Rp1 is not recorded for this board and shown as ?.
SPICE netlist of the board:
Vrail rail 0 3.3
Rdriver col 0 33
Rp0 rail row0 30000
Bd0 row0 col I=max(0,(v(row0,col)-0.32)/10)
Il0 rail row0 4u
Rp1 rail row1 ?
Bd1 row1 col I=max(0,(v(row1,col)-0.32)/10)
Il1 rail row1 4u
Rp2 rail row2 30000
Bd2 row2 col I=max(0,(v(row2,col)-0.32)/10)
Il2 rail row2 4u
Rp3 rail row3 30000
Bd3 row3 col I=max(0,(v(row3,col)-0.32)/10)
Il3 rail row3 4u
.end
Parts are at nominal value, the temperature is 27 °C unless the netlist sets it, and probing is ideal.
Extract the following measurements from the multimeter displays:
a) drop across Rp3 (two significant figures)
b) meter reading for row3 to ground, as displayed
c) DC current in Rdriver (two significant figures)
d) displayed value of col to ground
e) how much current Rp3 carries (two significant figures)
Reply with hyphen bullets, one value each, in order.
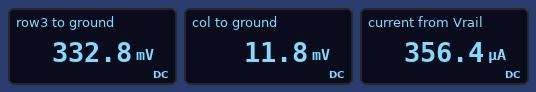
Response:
- 3.0 V
- 332.8 mV
- 360 µA
- 11.8 mV
- 99 µA
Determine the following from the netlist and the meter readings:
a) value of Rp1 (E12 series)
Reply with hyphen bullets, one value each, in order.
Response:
- 68 kΩ
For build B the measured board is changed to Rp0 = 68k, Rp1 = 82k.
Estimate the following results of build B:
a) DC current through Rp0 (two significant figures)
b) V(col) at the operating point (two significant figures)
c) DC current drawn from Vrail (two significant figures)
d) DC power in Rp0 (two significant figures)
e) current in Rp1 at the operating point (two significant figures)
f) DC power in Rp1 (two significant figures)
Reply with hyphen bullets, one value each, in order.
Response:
- 44 µA
- 9.7 mV
- 290 µA
- 130 µW
- 36 µA
- 110 µW
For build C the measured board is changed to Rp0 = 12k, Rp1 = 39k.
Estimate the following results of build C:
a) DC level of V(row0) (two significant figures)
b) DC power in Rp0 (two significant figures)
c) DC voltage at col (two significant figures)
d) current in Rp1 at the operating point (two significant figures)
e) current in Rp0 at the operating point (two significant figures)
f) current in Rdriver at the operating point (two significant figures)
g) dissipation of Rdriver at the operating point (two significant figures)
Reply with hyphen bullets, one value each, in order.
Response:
- 340 mV
- 730 µW
- 18 mV
- 76 µA
- 250 µA
- 540 µA
- 9.5 µW
